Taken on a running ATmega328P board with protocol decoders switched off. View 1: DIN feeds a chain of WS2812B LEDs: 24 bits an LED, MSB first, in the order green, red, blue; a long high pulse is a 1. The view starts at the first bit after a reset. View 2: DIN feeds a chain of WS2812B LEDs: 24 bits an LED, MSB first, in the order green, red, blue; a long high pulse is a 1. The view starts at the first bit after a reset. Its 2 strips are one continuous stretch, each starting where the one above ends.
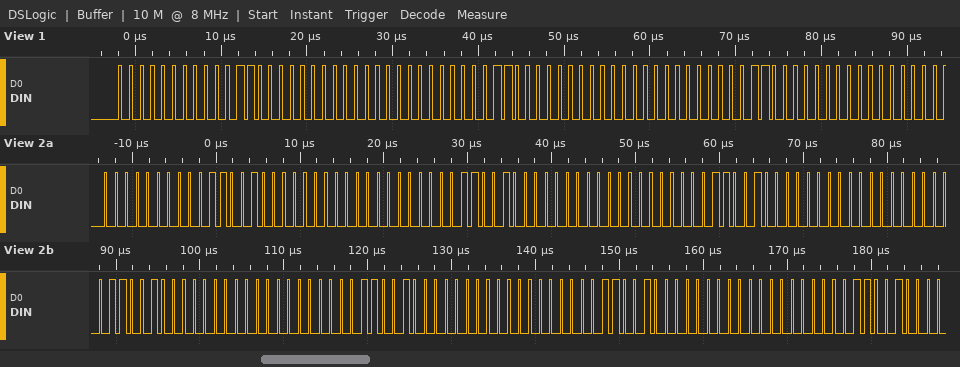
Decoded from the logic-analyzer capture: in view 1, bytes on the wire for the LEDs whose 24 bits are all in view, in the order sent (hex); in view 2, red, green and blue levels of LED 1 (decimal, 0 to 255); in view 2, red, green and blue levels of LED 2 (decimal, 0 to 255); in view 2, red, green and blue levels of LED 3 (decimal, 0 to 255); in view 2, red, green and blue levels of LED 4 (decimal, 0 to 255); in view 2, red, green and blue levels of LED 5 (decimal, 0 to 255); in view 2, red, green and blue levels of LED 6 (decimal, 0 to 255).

00 18 00 00 18 00 00 18 00
50, 0, 0
50, 0, 0
50, 0, 0
50, 0, 0
50, 0, 0
100, 0, 0
